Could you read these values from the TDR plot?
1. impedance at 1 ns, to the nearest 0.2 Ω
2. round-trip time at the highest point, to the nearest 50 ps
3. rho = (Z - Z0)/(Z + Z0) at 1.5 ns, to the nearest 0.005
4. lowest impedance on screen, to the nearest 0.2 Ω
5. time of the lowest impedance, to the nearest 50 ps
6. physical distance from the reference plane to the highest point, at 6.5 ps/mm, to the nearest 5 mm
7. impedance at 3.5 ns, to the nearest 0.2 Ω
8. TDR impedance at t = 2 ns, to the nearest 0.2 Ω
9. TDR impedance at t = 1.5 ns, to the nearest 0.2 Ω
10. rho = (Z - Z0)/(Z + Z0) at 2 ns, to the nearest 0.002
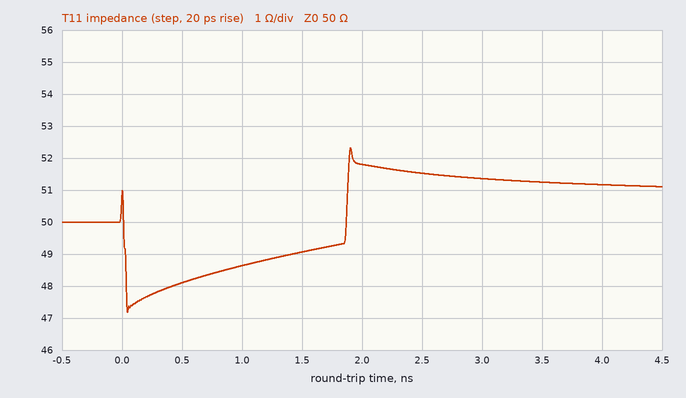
48.6 Ω
1.90 ns
-0.010
47.2 Ω
50 ps
145 mm
51.2 Ω
51.8 Ω
49.0 Ω
+0.018
